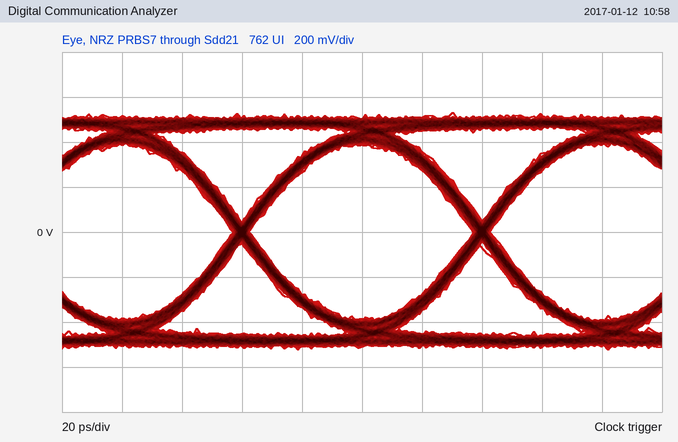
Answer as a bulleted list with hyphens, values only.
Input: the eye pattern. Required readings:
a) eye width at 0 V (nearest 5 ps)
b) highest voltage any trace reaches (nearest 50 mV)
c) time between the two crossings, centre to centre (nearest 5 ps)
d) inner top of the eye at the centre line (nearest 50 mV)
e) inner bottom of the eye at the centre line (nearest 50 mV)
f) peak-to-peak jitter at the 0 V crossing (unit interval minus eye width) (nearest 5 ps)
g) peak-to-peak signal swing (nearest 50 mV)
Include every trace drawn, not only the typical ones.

- 75 ps
- 550 mV
- 80 ps
- 400 mV
- -400 mV
- 5 ps
- 1.05 V
